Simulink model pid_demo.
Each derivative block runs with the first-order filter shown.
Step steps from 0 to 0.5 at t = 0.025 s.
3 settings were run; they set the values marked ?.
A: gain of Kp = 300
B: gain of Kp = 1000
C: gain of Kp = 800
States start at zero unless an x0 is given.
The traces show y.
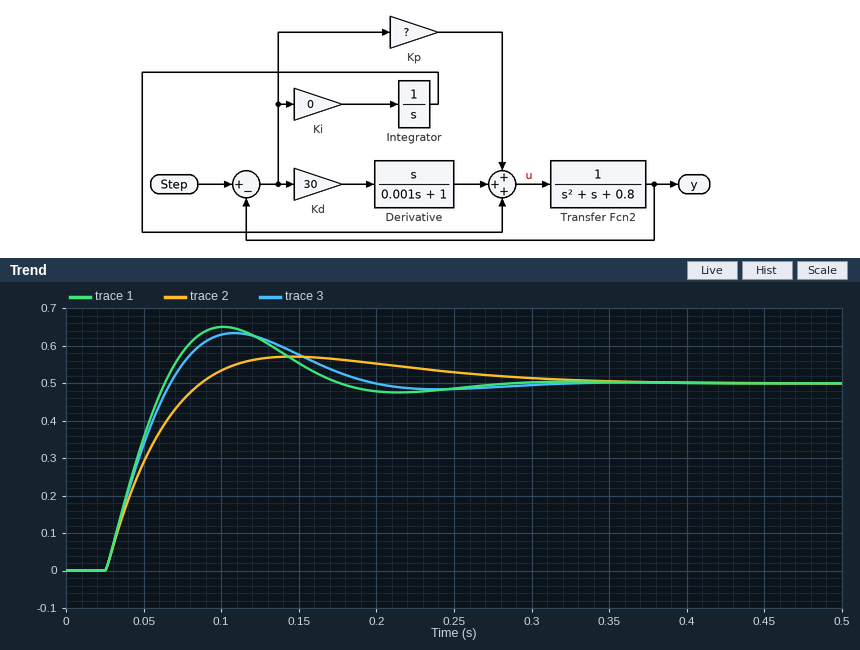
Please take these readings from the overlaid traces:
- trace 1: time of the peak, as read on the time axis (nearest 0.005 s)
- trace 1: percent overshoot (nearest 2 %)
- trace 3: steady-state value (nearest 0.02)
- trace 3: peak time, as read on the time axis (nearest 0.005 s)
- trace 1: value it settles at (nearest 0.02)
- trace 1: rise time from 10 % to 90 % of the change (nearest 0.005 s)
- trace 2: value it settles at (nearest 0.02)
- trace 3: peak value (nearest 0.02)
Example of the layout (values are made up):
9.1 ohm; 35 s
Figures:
0.100 s; 30 %; 0.50; 0.110 s; 0.50; 0.030 s; 0.50; 0.64
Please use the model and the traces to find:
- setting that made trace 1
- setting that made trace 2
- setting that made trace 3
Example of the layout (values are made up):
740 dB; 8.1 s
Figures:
B; A; C
